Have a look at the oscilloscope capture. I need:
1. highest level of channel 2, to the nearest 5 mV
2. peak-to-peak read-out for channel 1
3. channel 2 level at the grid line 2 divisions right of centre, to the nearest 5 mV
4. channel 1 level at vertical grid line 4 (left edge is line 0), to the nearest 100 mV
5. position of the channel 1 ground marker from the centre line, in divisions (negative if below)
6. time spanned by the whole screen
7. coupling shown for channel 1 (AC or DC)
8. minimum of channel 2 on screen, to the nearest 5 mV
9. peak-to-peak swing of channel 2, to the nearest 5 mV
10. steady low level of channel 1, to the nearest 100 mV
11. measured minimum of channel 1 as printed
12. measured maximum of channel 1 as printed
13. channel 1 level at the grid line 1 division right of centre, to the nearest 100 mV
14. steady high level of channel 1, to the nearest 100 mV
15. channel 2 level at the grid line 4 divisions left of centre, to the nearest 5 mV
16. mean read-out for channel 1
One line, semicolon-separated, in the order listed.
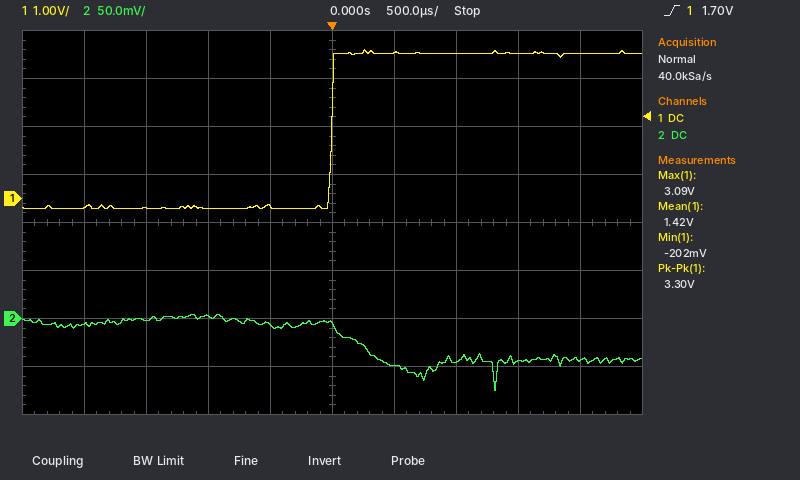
5 mV; 3.30 V; -45 mV; -200 mV; +0.5 div; 5 ms; DC; -75 mV; 80 mV; -200 mV; -202 mV; 3.09 V; 3.0 V; 3.0 V; -5 mV; 1.42 V
